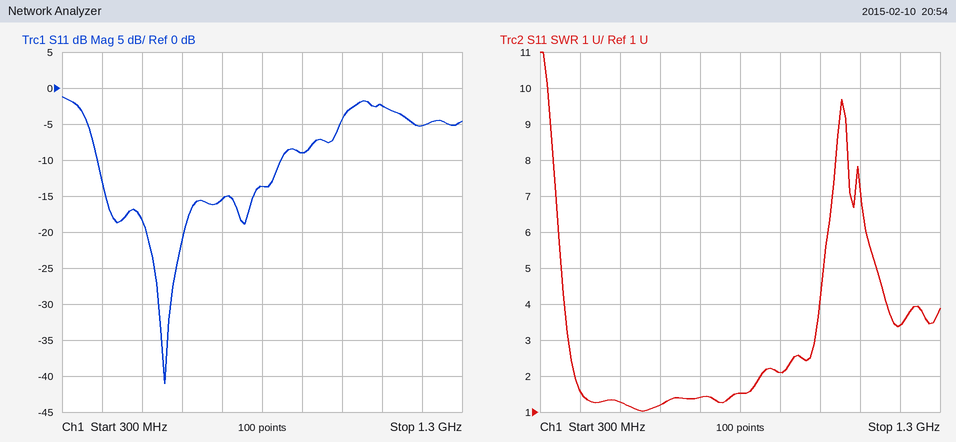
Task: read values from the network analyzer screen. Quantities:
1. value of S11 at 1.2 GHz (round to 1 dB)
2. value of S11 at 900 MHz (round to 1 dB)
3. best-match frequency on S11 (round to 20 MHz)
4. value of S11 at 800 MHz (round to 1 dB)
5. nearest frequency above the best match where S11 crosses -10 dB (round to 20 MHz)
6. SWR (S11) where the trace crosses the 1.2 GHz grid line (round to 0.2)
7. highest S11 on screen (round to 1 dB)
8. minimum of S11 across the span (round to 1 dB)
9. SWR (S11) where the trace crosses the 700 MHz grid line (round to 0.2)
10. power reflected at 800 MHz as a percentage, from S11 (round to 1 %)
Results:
-5 dB
-9 dB
560 MHz
-14 dB
840 MHz
3.4
-1 dB
-41 dB
1.4
4 %
